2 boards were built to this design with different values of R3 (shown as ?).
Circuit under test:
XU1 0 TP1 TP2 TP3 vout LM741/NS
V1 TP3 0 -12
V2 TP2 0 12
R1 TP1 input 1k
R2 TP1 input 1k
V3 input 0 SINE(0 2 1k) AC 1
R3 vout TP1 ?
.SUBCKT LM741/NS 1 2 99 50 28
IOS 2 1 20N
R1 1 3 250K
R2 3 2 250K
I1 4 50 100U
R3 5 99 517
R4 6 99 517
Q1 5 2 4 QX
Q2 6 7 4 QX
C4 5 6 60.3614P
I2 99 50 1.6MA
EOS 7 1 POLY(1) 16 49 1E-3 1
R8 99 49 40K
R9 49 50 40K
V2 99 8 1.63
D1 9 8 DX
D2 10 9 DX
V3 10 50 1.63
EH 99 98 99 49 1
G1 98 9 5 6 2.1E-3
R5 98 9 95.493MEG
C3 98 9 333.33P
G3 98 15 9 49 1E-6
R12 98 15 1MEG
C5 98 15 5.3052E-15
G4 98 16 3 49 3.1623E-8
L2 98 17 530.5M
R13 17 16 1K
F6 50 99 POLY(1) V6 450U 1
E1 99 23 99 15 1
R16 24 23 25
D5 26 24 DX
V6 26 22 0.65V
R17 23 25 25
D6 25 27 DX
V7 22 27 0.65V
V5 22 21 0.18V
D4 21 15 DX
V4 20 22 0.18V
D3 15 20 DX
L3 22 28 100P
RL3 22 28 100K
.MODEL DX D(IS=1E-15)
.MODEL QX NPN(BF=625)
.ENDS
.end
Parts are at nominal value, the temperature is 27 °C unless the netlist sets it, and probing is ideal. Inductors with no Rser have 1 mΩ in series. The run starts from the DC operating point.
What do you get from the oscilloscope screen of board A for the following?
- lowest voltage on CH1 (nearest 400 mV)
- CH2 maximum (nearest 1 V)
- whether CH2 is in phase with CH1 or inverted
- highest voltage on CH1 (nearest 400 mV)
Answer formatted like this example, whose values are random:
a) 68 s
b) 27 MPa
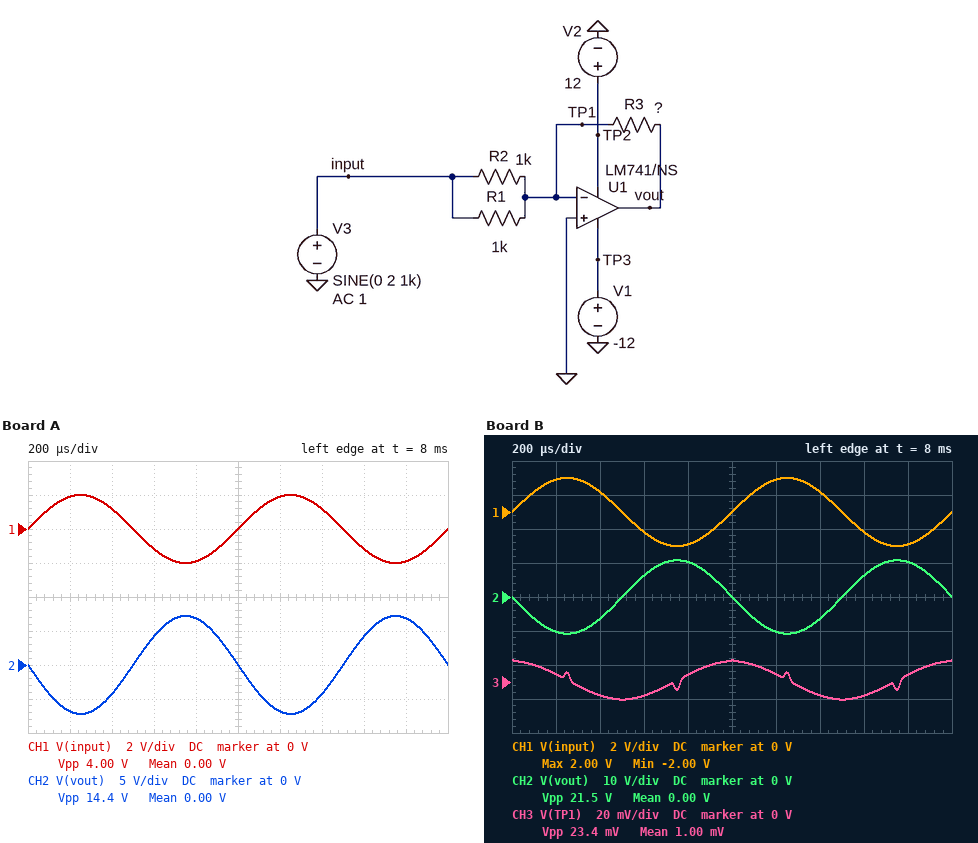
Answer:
a) -2.0 V
b) 7 V
c) inverted
d) 2.0 V
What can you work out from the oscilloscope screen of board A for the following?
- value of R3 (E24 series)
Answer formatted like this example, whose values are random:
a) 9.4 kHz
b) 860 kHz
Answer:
a) 1.8 kΩ
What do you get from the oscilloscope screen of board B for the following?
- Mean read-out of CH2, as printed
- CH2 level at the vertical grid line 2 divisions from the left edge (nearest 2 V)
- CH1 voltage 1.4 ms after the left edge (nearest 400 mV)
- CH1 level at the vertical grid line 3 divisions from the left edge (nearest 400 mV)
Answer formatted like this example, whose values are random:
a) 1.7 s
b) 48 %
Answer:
a) 0.00 V
b) -6 V
c) 1.2 V
d) -1.2 V
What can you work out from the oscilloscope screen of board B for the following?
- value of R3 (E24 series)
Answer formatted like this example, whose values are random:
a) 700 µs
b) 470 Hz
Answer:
a) 2.7 kΩ
